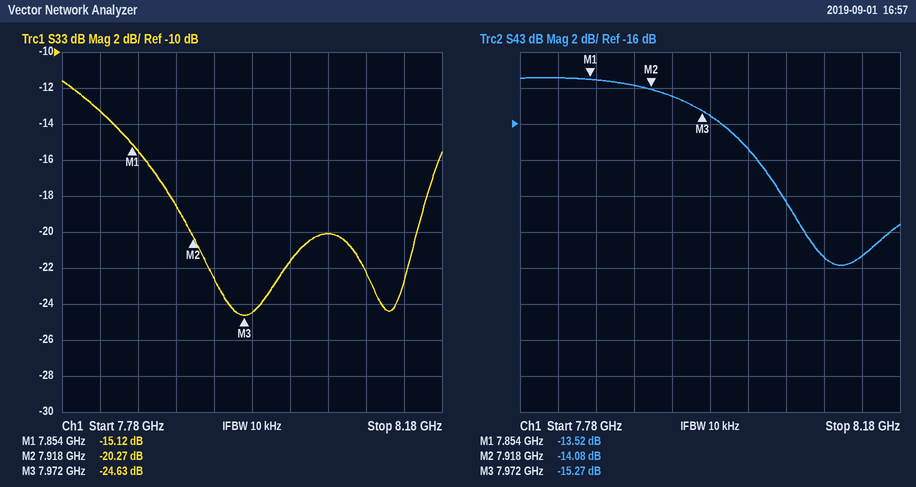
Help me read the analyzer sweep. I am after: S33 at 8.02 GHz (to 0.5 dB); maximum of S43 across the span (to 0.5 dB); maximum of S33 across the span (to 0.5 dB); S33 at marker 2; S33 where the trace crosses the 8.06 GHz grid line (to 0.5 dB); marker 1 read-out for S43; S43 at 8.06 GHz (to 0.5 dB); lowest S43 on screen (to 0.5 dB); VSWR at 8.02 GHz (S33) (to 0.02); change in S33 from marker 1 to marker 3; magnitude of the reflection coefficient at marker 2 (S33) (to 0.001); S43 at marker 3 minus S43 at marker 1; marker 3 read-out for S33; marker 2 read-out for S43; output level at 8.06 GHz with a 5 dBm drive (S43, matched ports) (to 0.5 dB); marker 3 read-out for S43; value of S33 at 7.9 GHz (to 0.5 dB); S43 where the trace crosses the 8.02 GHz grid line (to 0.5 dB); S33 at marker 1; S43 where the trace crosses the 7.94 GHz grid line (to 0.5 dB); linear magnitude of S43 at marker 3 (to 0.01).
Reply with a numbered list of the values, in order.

1. -21.5 dB
2. -13.5 dB
3. -11.5 dB
4. -20.27 dB
5. -20.0 dB
6. -13.52 dB
7. -20.5 dB
8. -24.0 dB
9. 1.18
10. -9.51 dB
11. 0.097
12. -1.75 dB
13. -24.63 dB
14. -14.08 dB
15. -15.5 dBm
16. -15.27 dB
17. -18.5 dB
18. -17.5 dB
19. -15.12 dB
20. -14.5 dB
21. 0.17
